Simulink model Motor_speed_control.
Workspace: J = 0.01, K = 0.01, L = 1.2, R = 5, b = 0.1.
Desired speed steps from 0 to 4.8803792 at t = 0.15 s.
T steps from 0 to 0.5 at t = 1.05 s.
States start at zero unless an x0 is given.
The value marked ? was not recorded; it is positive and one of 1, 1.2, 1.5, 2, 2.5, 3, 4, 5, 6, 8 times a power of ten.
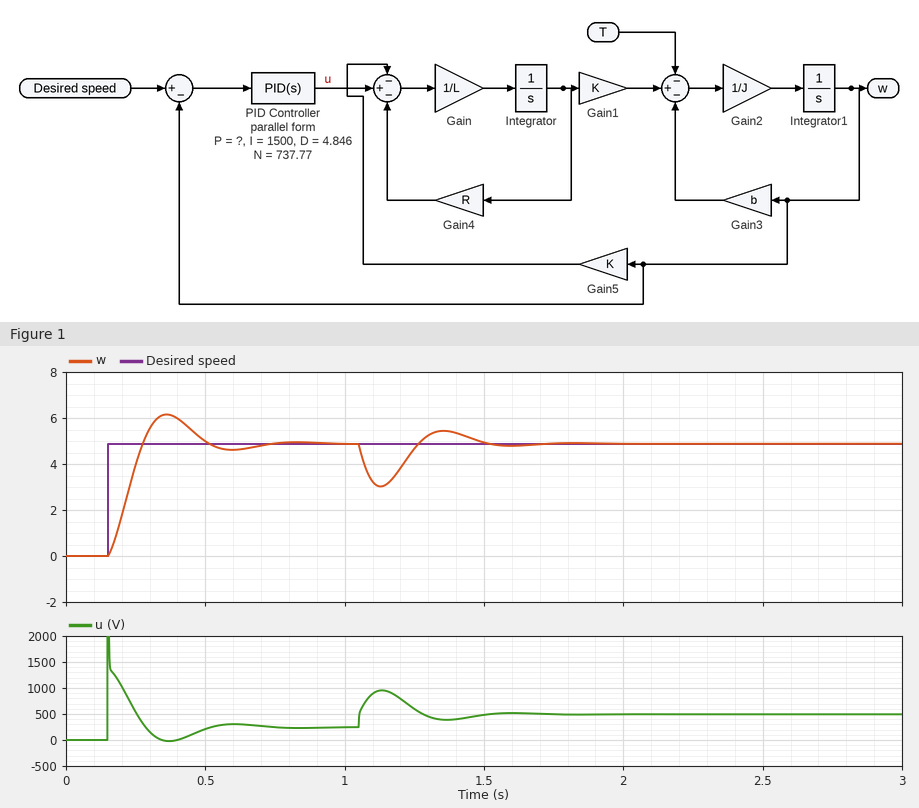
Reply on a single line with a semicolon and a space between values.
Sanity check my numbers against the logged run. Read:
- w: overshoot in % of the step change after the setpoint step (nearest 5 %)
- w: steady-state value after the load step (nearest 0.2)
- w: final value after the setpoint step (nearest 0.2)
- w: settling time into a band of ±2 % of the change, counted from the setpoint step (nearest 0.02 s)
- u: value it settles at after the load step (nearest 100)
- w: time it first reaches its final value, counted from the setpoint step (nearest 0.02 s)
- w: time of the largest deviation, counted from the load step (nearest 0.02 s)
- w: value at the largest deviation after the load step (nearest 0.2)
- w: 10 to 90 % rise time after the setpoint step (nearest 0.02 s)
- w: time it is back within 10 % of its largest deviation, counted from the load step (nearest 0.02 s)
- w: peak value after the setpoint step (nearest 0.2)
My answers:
25 %; 4.8; 4.8; 0.54 s; 500; 0.12 s; 0.08 s; 3.0; 0.10 s; 0.42 s; 6.2
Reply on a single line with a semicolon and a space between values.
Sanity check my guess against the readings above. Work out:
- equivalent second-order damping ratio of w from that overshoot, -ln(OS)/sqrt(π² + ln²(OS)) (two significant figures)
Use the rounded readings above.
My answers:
0.40
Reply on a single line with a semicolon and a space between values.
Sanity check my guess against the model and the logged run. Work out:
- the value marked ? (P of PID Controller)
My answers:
300
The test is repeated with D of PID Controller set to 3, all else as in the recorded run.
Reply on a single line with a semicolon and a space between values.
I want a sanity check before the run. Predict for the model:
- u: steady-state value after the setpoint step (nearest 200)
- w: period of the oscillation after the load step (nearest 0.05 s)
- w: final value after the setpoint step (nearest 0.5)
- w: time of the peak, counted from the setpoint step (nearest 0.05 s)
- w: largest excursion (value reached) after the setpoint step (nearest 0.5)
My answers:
200; 0.45 s; 5.0; 0.20 s; 6.5
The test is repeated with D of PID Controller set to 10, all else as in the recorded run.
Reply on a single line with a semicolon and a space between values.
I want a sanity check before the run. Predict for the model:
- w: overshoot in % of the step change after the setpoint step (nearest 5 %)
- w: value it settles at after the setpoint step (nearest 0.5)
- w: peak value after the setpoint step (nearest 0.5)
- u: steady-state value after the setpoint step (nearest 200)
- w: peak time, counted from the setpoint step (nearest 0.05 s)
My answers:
15 %; 5.0; 5.5; 200; 0.20 s
